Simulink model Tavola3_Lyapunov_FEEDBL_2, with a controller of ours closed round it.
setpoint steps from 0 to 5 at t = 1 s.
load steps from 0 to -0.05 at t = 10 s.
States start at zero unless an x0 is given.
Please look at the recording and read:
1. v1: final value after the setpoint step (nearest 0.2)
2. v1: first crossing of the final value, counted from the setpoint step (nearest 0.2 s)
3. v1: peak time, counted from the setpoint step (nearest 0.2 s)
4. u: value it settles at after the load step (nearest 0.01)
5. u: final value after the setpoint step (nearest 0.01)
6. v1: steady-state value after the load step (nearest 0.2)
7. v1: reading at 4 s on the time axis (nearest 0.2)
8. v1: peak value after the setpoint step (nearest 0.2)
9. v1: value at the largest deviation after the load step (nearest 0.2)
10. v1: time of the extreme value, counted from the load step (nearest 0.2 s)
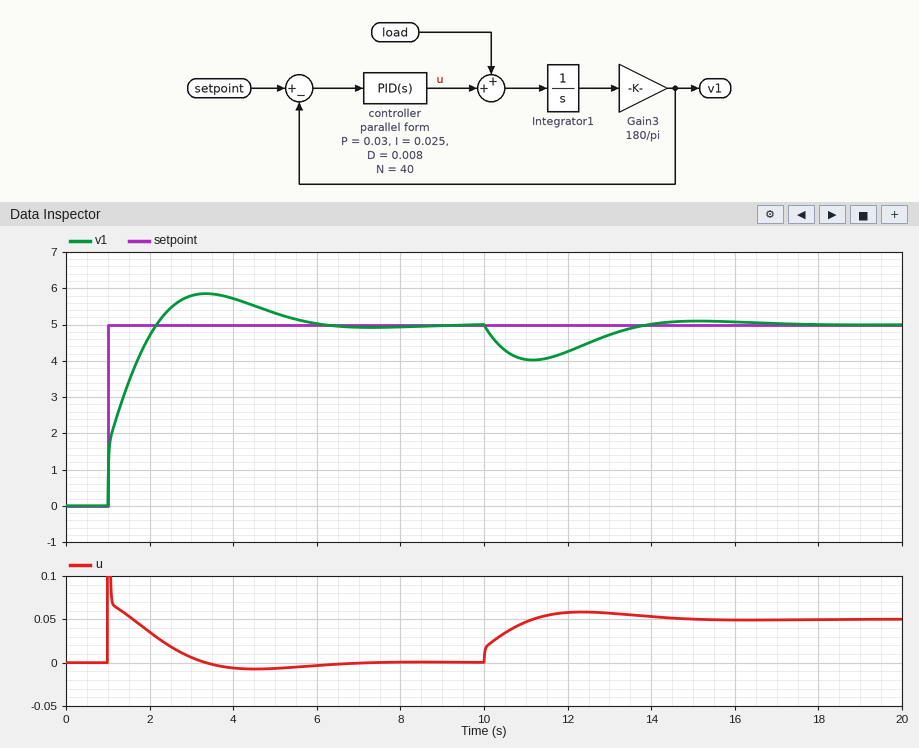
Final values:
5.0
1.2 s
2.4 s
0.05
0.00
5.0
5.8
5.8
4.0
1.2 s
